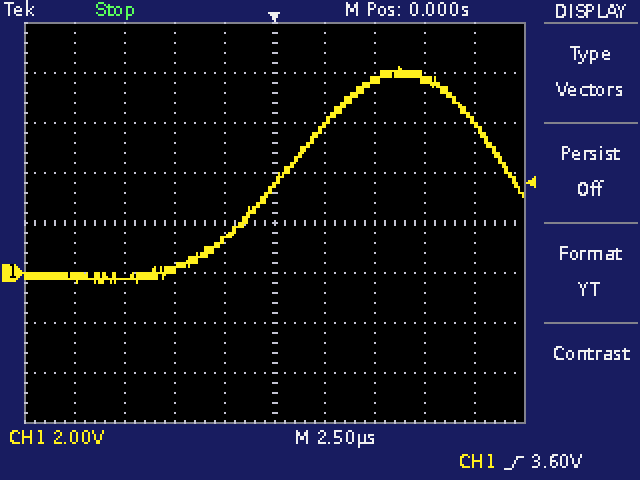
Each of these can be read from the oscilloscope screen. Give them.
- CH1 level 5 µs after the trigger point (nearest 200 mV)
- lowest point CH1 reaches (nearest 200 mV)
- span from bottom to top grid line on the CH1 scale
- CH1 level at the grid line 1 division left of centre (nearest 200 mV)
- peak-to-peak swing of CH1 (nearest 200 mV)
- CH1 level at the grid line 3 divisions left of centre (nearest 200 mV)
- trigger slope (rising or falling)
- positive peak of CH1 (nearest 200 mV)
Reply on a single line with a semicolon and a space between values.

7.8 V; -400 mV; 16 V; 1.4 V; 8.6 V; -200 mV; rising; 8.2 V
